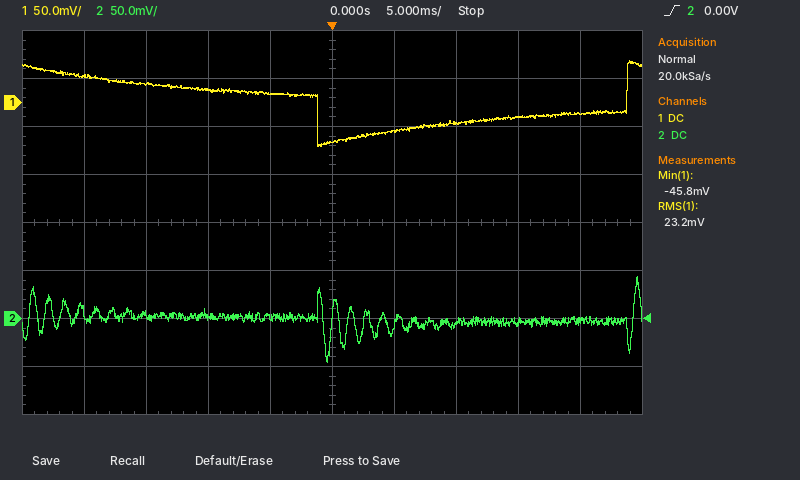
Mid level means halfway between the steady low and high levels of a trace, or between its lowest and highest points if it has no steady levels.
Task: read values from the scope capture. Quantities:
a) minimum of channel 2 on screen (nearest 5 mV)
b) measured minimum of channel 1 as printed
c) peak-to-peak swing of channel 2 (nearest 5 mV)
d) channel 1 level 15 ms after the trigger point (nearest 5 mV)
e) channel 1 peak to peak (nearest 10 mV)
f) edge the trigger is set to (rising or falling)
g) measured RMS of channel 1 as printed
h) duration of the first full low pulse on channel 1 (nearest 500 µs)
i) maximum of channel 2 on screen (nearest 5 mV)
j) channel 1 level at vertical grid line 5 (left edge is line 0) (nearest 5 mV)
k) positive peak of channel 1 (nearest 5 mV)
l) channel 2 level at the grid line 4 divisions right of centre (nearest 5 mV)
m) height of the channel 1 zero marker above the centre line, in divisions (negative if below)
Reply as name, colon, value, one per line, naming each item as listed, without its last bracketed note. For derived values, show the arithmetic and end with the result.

minimum of channel 2 on screen: -45 mV
measured minimum of channel 1 as printed: -45.8 mV
peak-to-peak swing of channel 2: 45 mV − (-45 mV) = 90 mV
channel 1 level 15 ms after the trigger point: -15 mV
channel 1 peak to peak: 90 mV
edge the trigger is set to: rising
measured RMS of channel 1 as printed: 23.2 mV
duration of the first full low pulse on channel 1: 25.0 ms
maximum of channel 2 on screen: 45 mV
channel 1 level at vertical grid line 5 (left edge is line 0): -40 mV
positive peak of channel 1: 45 mV
channel 2 level at the grid line 4 divisions right of centre: -5 mV
height of the channel 1 zero marker above the centre line, in divisions: +2.5 div
